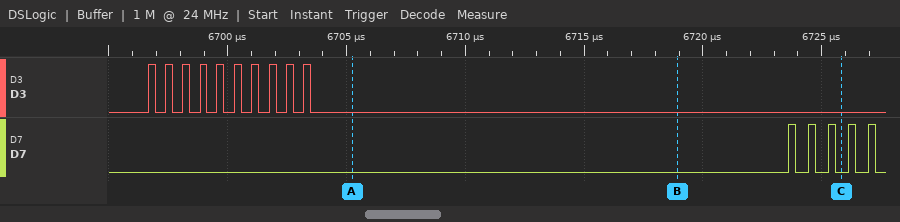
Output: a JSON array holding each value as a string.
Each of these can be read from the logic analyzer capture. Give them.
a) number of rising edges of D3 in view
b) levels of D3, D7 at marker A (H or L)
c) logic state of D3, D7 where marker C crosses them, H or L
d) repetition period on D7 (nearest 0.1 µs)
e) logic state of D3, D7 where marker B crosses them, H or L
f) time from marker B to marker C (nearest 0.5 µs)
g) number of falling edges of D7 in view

["10", "D3=L, D7=L", "D3=L, D7=L", "0.8 µs", "D3=L, D7=L", "7 µs", "5"]
